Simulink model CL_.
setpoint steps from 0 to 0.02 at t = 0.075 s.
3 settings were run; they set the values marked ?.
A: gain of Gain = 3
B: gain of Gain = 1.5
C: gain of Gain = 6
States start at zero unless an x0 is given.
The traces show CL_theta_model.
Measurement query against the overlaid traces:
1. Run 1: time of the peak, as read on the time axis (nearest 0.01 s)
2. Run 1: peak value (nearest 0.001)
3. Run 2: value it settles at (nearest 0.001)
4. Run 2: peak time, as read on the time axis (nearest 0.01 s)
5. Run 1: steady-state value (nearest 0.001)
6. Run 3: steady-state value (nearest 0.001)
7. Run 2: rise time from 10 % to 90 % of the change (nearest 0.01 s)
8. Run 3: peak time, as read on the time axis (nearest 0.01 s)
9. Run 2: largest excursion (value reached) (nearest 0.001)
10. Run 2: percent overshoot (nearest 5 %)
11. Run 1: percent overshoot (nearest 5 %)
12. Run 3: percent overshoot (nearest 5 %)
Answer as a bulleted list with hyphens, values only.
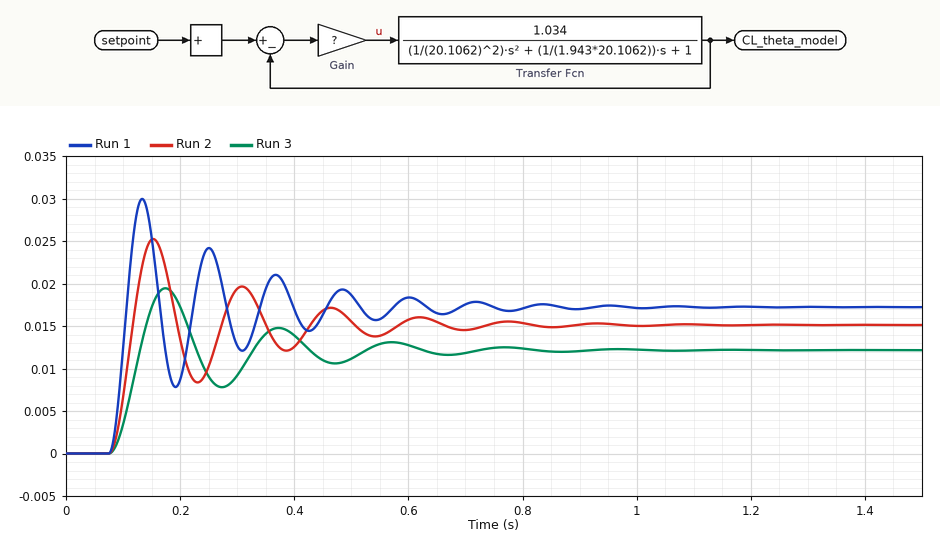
- 0.13 s
- 0.030
- 0.015
- 0.15 s
- 0.017
- 0.012
- 0.03 s
- 0.17 s
- 0.025
- 65 %
- 75 %
- 60 %
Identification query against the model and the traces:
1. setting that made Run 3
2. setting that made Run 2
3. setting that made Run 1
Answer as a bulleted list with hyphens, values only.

- B
- A
- C
